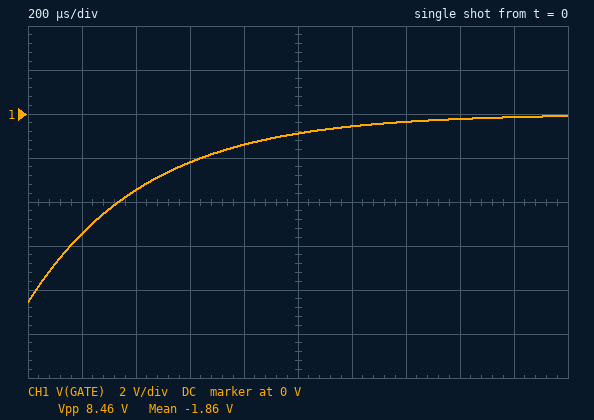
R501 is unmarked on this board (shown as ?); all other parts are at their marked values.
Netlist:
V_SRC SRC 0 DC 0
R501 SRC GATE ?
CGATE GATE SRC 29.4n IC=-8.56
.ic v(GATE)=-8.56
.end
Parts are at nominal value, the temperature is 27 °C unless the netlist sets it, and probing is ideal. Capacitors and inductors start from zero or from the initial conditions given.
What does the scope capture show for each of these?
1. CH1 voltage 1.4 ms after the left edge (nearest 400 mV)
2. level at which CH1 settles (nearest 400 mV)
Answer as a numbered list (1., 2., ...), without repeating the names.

1. -400 mV
2. 0 V
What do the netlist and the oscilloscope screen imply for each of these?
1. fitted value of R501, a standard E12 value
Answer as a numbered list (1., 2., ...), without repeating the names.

1. 15 kΩ
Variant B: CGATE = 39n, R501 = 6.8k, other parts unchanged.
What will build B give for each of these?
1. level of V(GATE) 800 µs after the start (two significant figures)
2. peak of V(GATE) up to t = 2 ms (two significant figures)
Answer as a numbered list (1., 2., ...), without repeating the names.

1. -420 mV
2. -4.5 mV
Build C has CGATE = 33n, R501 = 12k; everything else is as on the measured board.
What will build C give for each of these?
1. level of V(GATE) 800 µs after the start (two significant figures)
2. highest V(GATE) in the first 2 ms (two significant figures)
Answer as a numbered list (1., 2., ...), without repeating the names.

1. -1.1 V
2. -55 mV
